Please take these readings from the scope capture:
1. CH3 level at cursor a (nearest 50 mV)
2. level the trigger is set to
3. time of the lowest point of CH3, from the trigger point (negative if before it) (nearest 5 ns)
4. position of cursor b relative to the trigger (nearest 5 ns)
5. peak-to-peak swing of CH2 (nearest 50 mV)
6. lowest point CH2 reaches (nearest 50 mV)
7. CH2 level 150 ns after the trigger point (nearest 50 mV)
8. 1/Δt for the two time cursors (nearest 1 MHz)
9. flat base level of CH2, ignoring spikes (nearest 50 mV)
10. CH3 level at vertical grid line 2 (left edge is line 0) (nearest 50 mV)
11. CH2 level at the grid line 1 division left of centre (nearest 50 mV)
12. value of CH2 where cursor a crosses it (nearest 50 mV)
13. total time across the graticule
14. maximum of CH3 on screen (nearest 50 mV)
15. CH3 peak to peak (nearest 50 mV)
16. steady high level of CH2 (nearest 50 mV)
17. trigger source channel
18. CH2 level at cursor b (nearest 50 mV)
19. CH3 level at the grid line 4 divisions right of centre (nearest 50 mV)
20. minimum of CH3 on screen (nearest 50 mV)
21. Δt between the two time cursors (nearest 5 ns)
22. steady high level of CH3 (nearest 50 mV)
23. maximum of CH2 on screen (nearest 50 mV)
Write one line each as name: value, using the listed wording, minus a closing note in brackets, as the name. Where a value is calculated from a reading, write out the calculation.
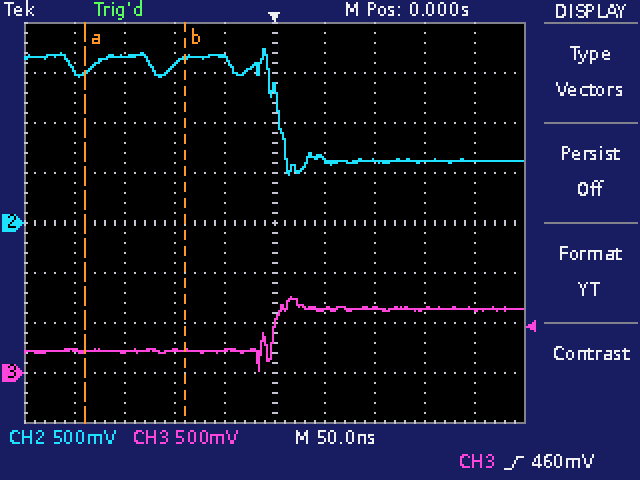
CH3 level at cursor a: 200 mV
level the trigger is set to: 460 mV
time of the lowest point of CH3, from the trigger point (negative if before it): -15 ns
position of cursor b relative to the trigger: -90 ns
peak-to-peak swing of CH2: 1.75 V − (500 mV) = 1.25 V
lowest point CH2 reaches: 500 mV
CH2 level 150 ns after the trigger point: 600 mV
1/Δt for the two time cursors: 1 / 100 ns ≈ 10 MHz
flat base level of CH2, ignoring spikes: 600 mV
CH3 level at vertical grid line 2 (left edge is line 0): 200 mV
CH2 level at the grid line 1 division left of centre: 1.65 V
value of CH2 where cursor a crosses it: 1.50 V
total time across the graticule: 500 ns
maximum of CH3 on screen: 750 mV
CH3 peak to peak: 750 mV − (0 mV) = 750 mV
steady high level of CH2: 1.65 V
trigger source channel: CH3
CH2 level at cursor b: 1.65 V
CH3 level at the grid line 4 divisions right of centre: 650 mV
minimum of CH3 on screen: 0 mV
Δt between the two time cursors: 100 ns
steady high level of CH3: 650 mV
maximum of CH2 on screen: 1.75 V
